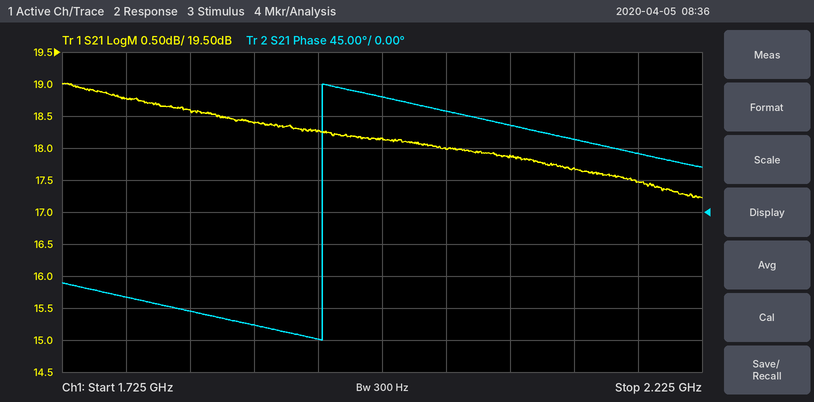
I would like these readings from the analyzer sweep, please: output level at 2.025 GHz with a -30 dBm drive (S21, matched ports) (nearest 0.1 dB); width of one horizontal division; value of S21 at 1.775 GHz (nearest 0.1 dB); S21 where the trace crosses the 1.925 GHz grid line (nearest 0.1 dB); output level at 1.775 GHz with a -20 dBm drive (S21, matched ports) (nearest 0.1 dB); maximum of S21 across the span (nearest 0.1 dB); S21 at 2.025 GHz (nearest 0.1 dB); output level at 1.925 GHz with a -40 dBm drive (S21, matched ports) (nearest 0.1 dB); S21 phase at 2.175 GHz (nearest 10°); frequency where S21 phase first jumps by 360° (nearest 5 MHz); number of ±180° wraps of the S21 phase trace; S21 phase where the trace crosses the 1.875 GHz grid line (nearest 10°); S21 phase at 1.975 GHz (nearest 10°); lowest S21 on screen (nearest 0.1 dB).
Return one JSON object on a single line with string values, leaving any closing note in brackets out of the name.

{"output level at 2.025 GHz with a -30 dBm drive (S21, matched ports)": "-12.0 dBm", "width of one horizontal division": "50 MHz", "value of S21 at 1.775 GHz": "18.8 dB", "S21 where the trace crosses the 1.925 GHz grid line": "18.3 dB", "output level at 1.775 GHz with a -20 dBm drive (S21, matched ports)": "-1.2 dBm", "maximum of S21 across the span": "19.0 dB", "S21 at 2.025 GHz": "18.0 dB", "output level at 1.925 GHz with a -40 dBm drive (S21, matched ports)": "-21.7 dBm", "S21 phase at 2.175 GHz": "80°", "frequency where S21 phase first jumps by 360°": "1.930 GHz", "number of ±180° wraps of the S21 phase trace": "1", "S21 phase where the trace crosses the 1.875 GHz grid line": "-160°", "S21 phase at 1.975 GHz": "160°", "lowest S21 on screen": "17.2 dB"}
